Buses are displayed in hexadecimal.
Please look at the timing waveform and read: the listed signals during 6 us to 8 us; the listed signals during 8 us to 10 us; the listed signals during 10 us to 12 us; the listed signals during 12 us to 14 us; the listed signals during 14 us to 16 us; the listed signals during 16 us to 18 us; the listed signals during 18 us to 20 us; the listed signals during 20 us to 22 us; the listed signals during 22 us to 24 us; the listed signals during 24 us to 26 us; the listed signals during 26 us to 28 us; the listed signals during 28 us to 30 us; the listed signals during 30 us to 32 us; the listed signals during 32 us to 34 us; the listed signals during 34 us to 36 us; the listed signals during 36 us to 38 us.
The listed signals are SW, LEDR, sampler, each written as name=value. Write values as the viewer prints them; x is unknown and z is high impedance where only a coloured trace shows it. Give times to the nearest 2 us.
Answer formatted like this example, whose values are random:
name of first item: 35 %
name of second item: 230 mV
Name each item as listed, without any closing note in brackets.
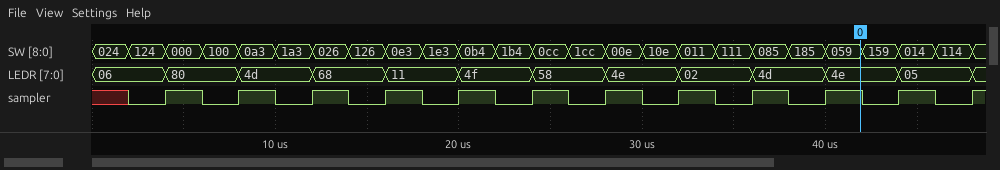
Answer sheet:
the listed signals during 6 us to 8 us: SW=100, LEDR=80, sampler=0
the listed signals during 8 us to 10 us: SW=0a3, LEDR=4d, sampler=1
the listed signals during 10 us to 12 us: SW=1a3, LEDR=4d, sampler=0
the listed signals during 12 us to 14 us: SW=026, LEDR=68, sampler=1
the listed signals during 14 us to 16 us: SW=126, LEDR=68, sampler=0
the listed signals during 16 us to 18 us: SW=0e3, LEDR=11, sampler=1
the listed signals during 18 us to 20 us: SW=1e3, LEDR=11, sampler=0
the listed signals during 20 us to 22 us: SW=0b4, LEDR=4f, sampler=1
the listed signals during 22 us to 24 us: SW=1b4, LEDR=4f, sampler=0
the listed signals during 24 us to 26 us: SW=0cc, LEDR=58, sampler=1
the listed signals during 26 us to 28 us: SW=1cc, LEDR=58, sampler=0
the listed signals during 28 us to 30 us: SW=00e, LEDR=4e, sampler=1
the listed signals during 30 us to 32 us: SW=10e, LEDR=4e, sampler=0
the listed signals during 32 us to 34 us: SW=011, LEDR=02, sampler=1
the listed signals during 34 us to 36 us: SW=111, LEDR=02, sampler=0
the listed signals during 36 us to 38 us: SW=085, LEDR=4d, sampler=1
